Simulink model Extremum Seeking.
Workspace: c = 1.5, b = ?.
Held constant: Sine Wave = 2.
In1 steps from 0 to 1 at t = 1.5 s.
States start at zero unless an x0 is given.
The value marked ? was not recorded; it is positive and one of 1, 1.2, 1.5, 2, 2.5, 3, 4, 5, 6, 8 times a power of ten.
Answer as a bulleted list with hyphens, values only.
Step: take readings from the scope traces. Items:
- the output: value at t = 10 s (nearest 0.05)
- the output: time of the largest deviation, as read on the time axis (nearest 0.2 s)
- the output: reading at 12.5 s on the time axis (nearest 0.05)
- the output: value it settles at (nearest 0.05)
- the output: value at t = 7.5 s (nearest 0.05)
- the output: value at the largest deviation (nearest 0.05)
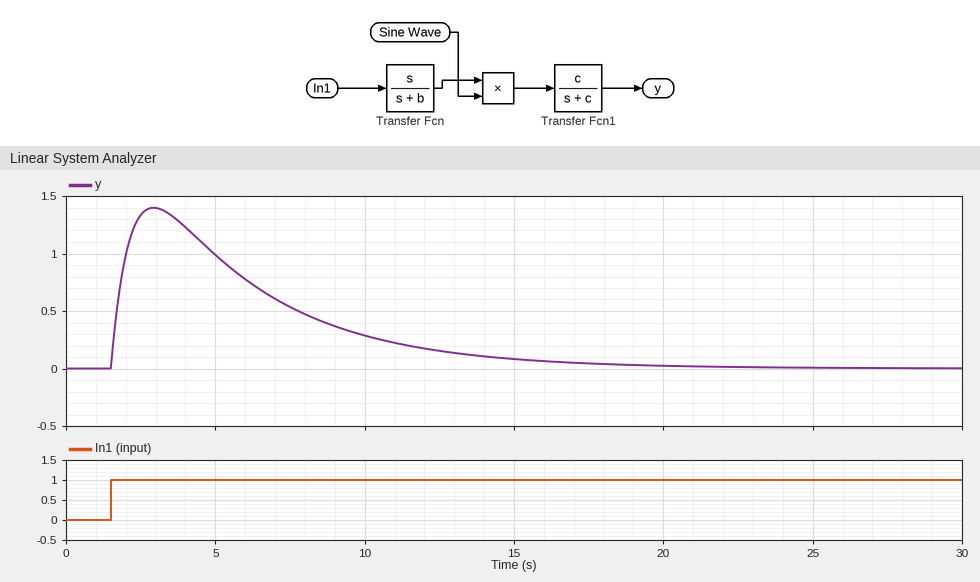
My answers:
- 0.30
- 3.0 s
- 0.15
- 0.00
- 0.55
- 1.40
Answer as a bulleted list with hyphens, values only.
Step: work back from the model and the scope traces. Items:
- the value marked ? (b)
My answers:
- 0.25
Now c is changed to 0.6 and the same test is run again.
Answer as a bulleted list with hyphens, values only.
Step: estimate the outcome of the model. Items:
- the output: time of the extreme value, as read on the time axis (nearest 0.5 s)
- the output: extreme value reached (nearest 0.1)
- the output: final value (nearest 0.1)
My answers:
- 4.0 s
- 1.1
- 0.0
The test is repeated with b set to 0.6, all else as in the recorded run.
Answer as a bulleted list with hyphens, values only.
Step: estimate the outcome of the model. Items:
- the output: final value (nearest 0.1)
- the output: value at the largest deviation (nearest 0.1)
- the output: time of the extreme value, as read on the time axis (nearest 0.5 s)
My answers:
- 0.0
- 1.1
- 2.5 s
